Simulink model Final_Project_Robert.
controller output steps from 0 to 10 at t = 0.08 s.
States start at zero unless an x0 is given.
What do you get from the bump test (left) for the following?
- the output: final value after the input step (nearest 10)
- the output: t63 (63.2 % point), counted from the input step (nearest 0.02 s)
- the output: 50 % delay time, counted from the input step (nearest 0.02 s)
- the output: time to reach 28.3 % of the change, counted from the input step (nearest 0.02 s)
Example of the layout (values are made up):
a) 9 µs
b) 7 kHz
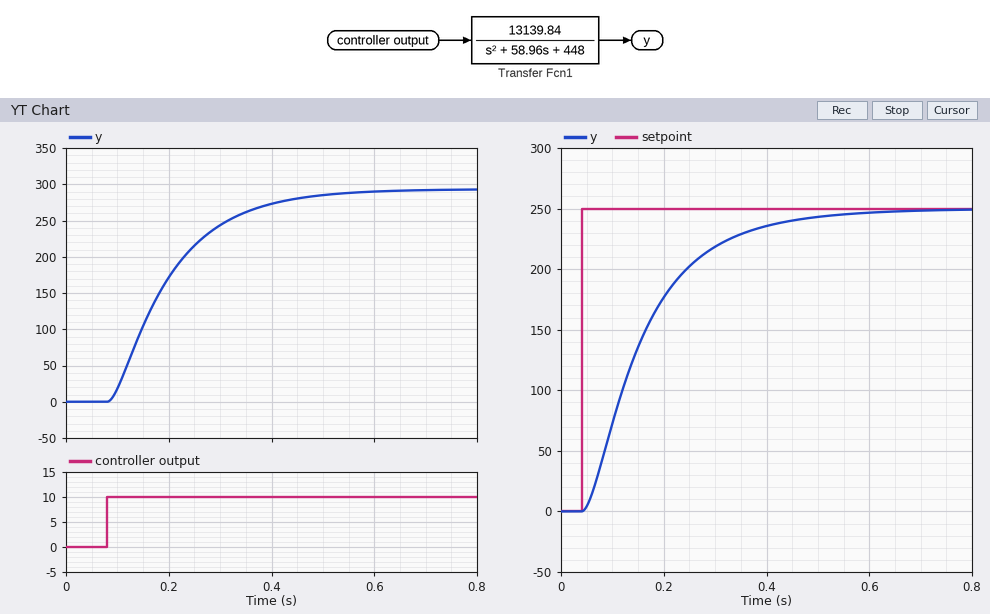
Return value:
a) 290
b) 0.14 s
c) 0.10 s
d) 0.06 s
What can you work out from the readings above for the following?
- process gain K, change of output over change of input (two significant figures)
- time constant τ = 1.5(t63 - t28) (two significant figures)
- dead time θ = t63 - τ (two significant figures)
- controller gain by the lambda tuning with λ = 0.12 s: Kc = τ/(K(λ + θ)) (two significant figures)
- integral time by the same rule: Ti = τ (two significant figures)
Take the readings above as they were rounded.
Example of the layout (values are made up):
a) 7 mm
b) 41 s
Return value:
a) 29
b) 0.12 s
c) 0.020 s
d) 0.030
e) 0.12 s
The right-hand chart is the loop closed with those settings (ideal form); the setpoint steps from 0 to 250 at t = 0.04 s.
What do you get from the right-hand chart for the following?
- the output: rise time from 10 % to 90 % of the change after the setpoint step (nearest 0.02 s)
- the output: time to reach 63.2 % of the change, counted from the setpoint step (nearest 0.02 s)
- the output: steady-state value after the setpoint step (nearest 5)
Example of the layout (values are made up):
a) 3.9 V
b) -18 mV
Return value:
a) 0.26 s
b) 0.14 s
c) 250
